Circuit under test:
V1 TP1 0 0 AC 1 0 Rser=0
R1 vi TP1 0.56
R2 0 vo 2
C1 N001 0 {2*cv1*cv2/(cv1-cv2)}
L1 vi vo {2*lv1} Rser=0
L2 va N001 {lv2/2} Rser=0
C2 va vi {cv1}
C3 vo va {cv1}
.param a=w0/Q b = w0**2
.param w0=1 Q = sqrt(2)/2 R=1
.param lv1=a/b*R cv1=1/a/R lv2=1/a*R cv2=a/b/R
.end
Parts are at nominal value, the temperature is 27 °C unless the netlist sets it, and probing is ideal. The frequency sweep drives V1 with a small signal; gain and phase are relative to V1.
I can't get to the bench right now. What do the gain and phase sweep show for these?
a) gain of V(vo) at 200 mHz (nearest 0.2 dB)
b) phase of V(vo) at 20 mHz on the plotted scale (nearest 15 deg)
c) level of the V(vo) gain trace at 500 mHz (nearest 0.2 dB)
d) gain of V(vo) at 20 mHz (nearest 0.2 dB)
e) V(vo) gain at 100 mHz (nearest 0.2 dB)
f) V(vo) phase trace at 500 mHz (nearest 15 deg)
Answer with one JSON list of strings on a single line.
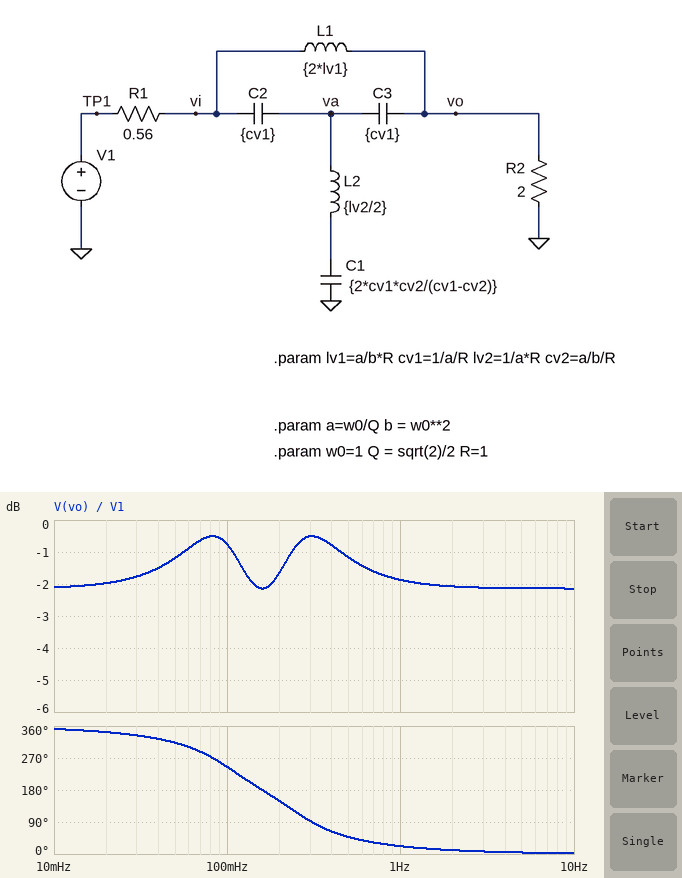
["-1.6 dB", "345 deg", "-1.2 dB", "-2.0 dB", "-0.8 dB", "45 deg"]
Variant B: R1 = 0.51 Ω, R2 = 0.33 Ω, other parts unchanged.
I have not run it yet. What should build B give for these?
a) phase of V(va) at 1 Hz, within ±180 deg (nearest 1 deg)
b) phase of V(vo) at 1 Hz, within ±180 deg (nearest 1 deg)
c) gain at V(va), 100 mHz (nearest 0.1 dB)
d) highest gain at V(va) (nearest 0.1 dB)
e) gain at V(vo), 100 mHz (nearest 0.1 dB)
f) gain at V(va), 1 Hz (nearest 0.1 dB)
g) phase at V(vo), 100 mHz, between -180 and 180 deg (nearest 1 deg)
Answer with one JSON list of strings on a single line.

["-1 deg", "34 deg", "-0.2 dB", "4.5 dB", "-10.7 dB", "-7.1 dB", "-106 deg"]
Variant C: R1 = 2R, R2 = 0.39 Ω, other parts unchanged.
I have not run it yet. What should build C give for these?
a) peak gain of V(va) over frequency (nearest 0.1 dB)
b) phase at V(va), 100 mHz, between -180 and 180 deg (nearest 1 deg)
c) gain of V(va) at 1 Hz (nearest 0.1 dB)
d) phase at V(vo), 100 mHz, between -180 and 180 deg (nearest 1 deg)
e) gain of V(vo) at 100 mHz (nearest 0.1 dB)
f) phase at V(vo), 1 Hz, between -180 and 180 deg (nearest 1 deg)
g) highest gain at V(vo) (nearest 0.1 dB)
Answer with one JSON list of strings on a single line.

["-4.4 dB", "137 deg", "-14.1 dB", "-118 deg", "-13.6 dB", "20 deg", "-13.2 dB"]
